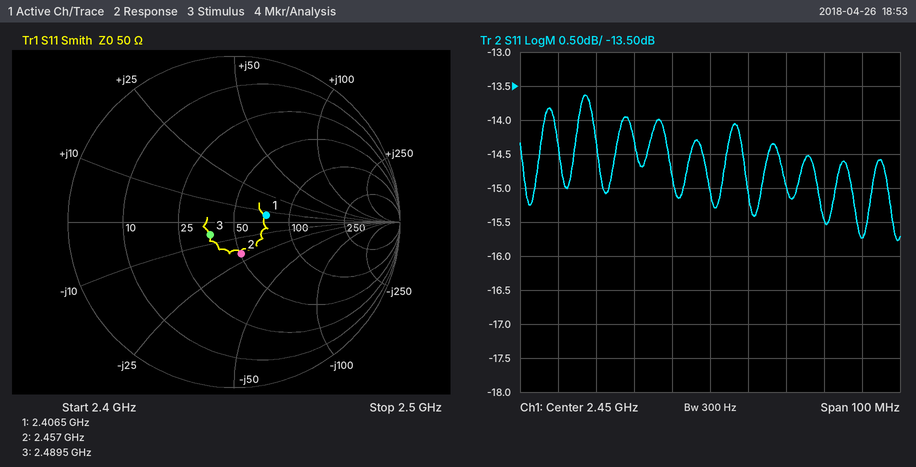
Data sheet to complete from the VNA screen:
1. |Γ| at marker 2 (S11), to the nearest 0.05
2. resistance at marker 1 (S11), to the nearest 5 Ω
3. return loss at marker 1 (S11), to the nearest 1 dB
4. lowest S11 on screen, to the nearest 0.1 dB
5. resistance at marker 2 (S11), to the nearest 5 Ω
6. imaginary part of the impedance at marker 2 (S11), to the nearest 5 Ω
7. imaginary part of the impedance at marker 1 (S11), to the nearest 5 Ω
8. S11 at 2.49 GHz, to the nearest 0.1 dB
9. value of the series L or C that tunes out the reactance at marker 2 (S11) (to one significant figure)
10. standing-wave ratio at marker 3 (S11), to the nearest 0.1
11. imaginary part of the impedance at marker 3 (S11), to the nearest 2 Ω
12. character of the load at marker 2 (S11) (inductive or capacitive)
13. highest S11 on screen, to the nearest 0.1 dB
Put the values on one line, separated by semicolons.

0.20; 75 Ω; 14 dB; -15.8 dB; 50 Ω; -20 Ω; +5 Ω; -15.7 dB; 1 nH; 1.4; -6 Ω; capacitive; -13.6 dB
